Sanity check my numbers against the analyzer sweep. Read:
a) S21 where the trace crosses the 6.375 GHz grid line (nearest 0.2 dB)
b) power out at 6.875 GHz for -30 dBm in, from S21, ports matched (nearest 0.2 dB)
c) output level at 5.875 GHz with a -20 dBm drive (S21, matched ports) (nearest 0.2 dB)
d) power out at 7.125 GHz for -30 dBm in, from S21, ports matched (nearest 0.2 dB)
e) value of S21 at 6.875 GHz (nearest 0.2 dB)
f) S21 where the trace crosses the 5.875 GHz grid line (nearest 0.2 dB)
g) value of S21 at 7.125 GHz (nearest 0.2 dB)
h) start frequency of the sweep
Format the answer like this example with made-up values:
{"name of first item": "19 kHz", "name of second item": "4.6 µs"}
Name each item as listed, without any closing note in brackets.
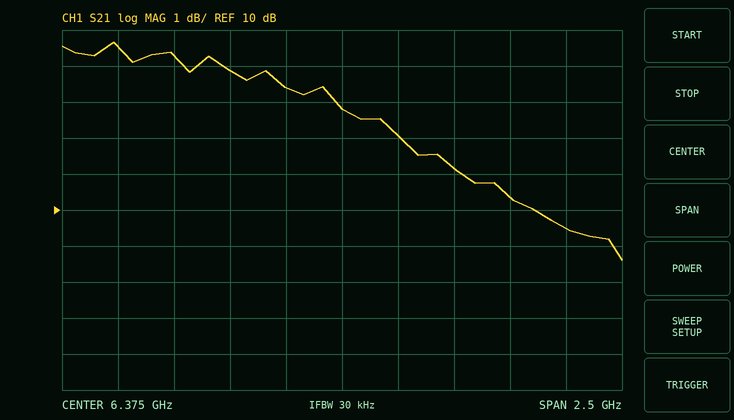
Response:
{"S21 where the trace crosses the 6.375 GHz grid line": "12.8 dB", "power out at 6.875 GHz for -30 dBm in, from S21, ports matched": "-18.8 dBm", "output level at 5.875 GHz with a -20 dBm drive (S21, matched ports)": "-6.2 dBm", "power out at 7.125 GHz for -30 dBm in, from S21, ports matched": "-19.6 dBm", "value of S21 at 6.875 GHz": "11.2 dB", "S21 where the trace crosses the 5.875 GHz grid line": "13.8 dB", "value of S21 at 7.125 GHz": "10.4 dB", "start frequency of the sweep": "5.125 GHz"}
